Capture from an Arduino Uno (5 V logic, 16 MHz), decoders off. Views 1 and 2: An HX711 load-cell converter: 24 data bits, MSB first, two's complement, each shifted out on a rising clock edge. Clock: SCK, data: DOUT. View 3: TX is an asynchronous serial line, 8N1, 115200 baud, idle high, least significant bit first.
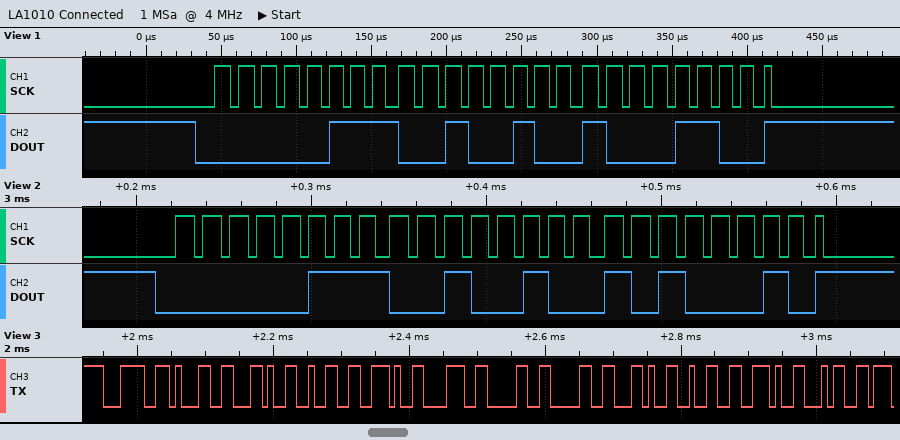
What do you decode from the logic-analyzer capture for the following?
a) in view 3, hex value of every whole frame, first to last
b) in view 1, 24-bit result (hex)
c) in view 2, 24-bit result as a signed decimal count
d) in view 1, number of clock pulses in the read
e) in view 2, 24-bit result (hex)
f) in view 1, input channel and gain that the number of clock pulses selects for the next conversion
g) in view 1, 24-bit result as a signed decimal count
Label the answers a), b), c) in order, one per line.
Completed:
a) 0x3C 0x31 0x2C 0x32 0x2E 0x38 0x30 0x30 0x2C 0x32 0x2E 0x34
b) 0x07248C
c) 468130
d) 25
e) 0x0724A2
f) channel A, gain 128
g) 468108
